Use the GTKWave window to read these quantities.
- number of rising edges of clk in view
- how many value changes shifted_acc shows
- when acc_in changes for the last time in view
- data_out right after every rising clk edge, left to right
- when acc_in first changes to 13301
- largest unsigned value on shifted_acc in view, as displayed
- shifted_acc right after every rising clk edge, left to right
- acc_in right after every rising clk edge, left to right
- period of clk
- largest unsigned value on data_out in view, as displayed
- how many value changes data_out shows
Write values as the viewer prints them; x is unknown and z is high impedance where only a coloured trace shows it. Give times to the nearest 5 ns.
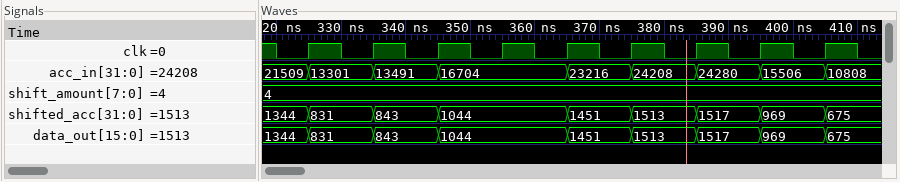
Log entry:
9
8
405 ns
831, 843, 1044, 1044, 1451, 1513, 1517, 969, 675
325 ns
1517
831, 843, 1044, 1044, 1451, 1513, 1517, 969, 675
13301, 13491, 16704, 16704, 23216, 24208, 24280, 15506, 10808
10 ns
1517
8
